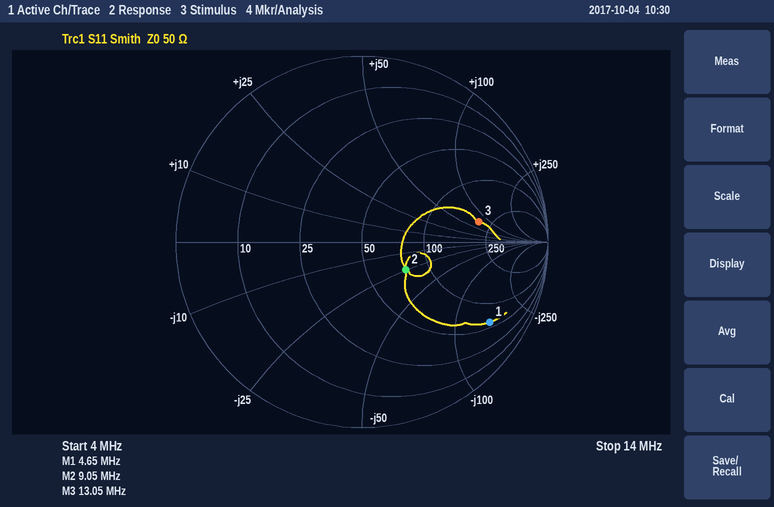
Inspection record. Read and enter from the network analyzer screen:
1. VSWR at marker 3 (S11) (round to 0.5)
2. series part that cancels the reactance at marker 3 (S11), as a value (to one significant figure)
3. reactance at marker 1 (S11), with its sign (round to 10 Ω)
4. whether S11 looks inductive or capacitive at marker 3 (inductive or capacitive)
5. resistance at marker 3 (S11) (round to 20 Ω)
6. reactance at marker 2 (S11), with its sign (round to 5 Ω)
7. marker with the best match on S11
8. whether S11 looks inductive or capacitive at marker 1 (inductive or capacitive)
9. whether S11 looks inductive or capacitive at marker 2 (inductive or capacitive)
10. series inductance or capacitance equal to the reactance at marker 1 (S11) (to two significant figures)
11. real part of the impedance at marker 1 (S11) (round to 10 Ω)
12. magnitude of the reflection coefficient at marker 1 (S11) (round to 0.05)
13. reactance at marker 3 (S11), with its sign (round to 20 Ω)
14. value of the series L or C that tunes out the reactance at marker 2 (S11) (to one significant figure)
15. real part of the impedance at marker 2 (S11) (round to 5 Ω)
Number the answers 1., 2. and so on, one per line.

1. 4.5
2. 200 pF
3. -150 Ω
4. inductive
5. 200 Ω
6. -25 Ω
7. marker 2
8. capacitive
9. capacitive
10. 230 pF
11. 60 Ω
12. 0.80
13. +80 Ω
14. 400 nH
15. 75 Ω
